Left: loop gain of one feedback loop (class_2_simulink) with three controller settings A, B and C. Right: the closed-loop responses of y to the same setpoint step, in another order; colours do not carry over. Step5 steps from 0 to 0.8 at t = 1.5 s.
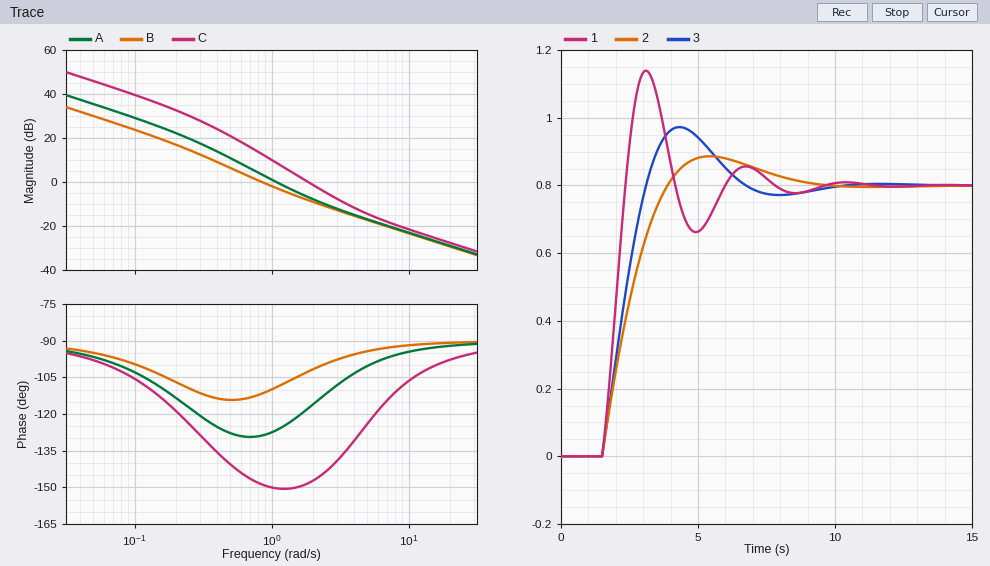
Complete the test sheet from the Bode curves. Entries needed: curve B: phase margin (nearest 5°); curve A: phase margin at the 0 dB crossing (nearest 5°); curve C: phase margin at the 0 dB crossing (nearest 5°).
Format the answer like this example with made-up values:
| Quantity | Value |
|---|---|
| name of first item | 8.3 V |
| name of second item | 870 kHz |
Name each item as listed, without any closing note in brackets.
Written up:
| Quantity | Value |
|---|---|
| curve B: phase margin | 70° |
| curve A: phase margin at the 0 dB crossing | 55° |
| curve C: phase margin at the 0 dB crossing | 30° |
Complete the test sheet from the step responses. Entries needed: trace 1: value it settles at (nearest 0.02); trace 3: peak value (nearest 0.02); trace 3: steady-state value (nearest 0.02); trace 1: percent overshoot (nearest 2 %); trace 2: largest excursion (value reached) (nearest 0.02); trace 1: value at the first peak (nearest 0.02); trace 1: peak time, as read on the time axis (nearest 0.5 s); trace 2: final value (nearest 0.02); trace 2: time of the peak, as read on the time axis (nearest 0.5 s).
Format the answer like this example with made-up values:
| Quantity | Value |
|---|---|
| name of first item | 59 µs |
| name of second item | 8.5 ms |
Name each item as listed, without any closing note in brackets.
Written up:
| Quantity | Value |
|---|---|
| trace 1: value it settles at | 0.80 |
| trace 3: peak value | 0.98 |
| trace 3: steady-state value | 0.80 |
| trace 1: percent overshoot | 42 % |
| trace 2: largest excursion (value reached) | 0.88 |
| trace 1: value at the first peak | 1.14 |
| trace 1: peak time, as read on the time axis | 3.0 s |
| trace 2: final value | 0.80 |
| trace 2: time of the peak, as read on the time axis | 5.5 s |
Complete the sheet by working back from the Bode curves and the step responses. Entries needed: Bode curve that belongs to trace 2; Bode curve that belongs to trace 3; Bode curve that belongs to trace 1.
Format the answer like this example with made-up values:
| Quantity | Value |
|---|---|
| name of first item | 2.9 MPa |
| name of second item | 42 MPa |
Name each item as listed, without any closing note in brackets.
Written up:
| Quantity | Value |
|---|---|
| Bode curve that belongs to trace 2 | B |
| Bode curve that belongs to trace 3 | A |
| Bode curve that belongs to trace 1 | C |
